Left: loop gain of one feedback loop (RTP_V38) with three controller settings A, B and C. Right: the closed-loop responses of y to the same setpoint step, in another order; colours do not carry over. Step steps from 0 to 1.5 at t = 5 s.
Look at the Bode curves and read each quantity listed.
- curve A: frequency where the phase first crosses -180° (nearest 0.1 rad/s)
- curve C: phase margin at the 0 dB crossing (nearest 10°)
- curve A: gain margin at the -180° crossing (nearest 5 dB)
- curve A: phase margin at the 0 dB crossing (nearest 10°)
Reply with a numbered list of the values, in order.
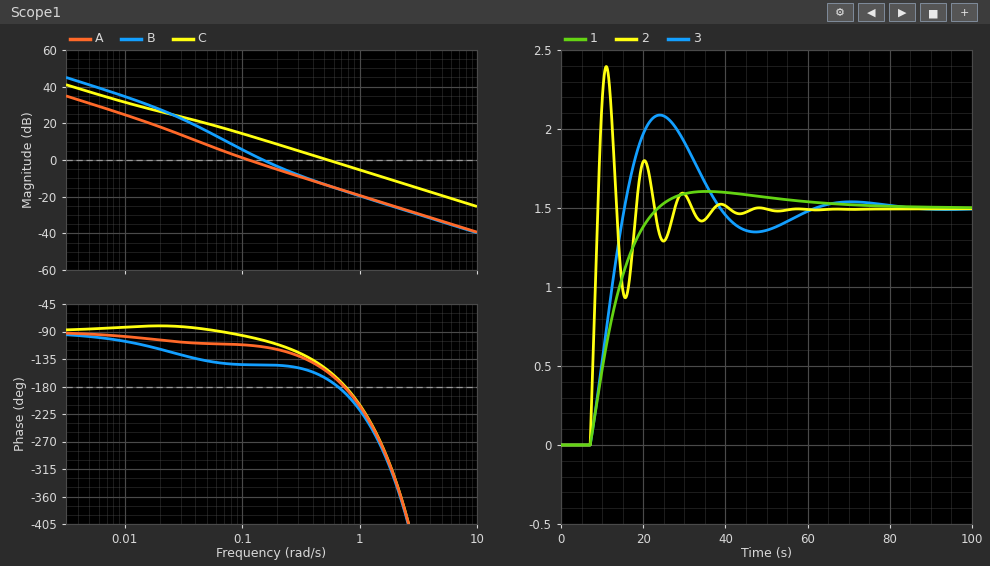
1. 0.7 rad/s
2. 30°
3. 15 dB
4. 70°
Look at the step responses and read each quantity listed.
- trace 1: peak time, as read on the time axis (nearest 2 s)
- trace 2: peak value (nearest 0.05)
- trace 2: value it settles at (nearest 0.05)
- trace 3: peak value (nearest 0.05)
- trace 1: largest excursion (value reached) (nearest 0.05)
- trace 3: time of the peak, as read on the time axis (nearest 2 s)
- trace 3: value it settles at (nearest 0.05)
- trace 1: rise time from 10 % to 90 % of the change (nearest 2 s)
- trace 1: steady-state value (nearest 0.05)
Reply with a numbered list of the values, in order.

1. 36 s
2. 2.40
3. 1.50
4. 2.10
5. 1.60
6. 24 s
7. 1.50
8. 12 s
9. 1.50
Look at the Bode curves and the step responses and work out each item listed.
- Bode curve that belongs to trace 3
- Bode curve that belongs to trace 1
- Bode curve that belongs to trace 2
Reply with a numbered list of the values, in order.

1. B
2. A
3. C
